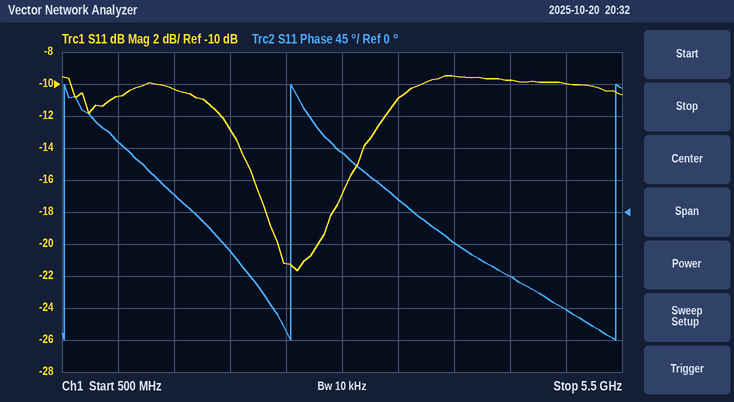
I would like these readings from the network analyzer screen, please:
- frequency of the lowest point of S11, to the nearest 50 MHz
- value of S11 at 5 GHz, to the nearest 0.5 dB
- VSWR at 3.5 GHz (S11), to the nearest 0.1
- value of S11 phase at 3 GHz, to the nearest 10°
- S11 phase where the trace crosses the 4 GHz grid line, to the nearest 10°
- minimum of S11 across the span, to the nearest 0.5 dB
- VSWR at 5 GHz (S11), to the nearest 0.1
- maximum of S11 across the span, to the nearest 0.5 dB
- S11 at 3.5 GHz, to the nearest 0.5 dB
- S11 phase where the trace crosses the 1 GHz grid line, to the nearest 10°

2.60 GHz
-10.0 dB
1.8
80°
-40°
-21.5 dB
1.9
-9.5 dB
-11.0 dB
100°
